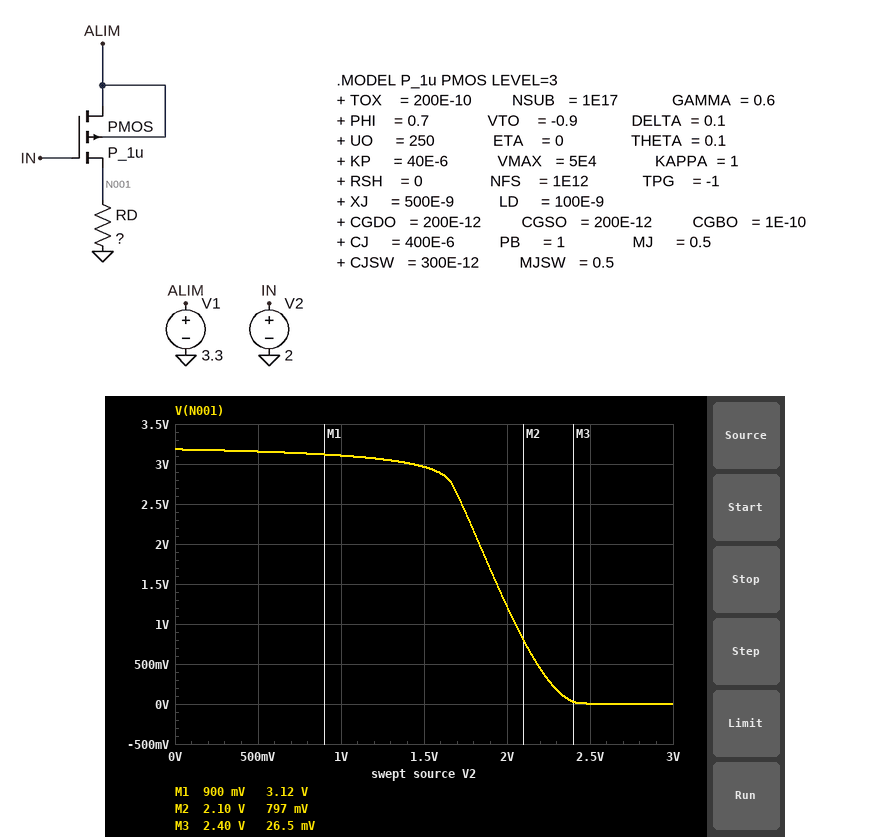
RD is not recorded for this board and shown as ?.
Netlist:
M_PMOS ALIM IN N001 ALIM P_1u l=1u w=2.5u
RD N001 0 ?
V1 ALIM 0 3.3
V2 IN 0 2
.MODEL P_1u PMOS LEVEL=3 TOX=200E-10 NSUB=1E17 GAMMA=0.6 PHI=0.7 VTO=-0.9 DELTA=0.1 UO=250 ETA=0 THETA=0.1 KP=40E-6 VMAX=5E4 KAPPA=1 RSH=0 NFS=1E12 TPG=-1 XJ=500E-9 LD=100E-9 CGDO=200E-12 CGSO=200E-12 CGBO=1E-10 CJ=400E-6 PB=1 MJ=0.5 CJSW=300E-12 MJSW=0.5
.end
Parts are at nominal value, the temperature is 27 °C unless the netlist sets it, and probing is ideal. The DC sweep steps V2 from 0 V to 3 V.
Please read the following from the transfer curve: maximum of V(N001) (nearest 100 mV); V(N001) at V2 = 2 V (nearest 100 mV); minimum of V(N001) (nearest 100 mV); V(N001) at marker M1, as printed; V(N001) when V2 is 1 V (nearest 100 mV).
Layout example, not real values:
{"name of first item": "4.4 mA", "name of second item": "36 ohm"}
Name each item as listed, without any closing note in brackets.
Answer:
{"maximum of V(N001)": "3.2 V", "V(N001) at V2 = 2 V": "1.2 V", "minimum of V(N001)": "0 V", "V(N001) at marker M1, as printed": "3.12 V", "V(N001) when V2 is 1 V": "3.1 V"}
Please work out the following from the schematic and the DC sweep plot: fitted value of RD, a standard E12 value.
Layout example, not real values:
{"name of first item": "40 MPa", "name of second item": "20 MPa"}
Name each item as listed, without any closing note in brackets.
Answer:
{"fitted value of RD, a standard E12 value": "120 kΩ"}
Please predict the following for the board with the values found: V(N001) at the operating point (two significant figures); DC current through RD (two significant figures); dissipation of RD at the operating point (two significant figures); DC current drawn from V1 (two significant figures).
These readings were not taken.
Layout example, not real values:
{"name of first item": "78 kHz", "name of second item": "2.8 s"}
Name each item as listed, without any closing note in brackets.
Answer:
{"V(N001) at the operating point": "1.2 V", "DC current through RD": "10 µA", "dissipation of RD at the operating point": "12 µW", "DC current drawn from V1": "10 µA"}
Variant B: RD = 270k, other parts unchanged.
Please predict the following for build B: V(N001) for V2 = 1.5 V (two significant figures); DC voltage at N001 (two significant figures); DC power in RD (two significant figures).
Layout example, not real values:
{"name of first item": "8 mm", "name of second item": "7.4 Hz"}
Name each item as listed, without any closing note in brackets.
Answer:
{"V(N001) for V2 = 1.5 V": "3.2 V", "DC voltage at N001": "2.5 V", "DC power in RD": "24 µW"}
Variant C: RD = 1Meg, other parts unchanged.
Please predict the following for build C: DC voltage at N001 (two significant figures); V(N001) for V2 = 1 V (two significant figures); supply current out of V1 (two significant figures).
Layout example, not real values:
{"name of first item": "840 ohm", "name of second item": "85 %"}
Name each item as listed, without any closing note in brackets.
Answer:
{"DC voltage at N001": "3.2 V", "V(N001) for V2 = 1 V": "3.3 V", "supply current out of V1": "3.2 µA"}
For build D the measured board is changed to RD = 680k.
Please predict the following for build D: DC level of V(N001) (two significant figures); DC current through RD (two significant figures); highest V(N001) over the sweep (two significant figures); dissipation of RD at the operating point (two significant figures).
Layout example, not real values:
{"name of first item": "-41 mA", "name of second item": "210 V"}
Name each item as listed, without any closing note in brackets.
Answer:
{"DC level of V(N001)": "3.2 V", "DC current through RD": "4.7 µA", "highest V(N001) over the sweep": "3.3 V", "dissipation of RD at the operating point": "15 µW"}
